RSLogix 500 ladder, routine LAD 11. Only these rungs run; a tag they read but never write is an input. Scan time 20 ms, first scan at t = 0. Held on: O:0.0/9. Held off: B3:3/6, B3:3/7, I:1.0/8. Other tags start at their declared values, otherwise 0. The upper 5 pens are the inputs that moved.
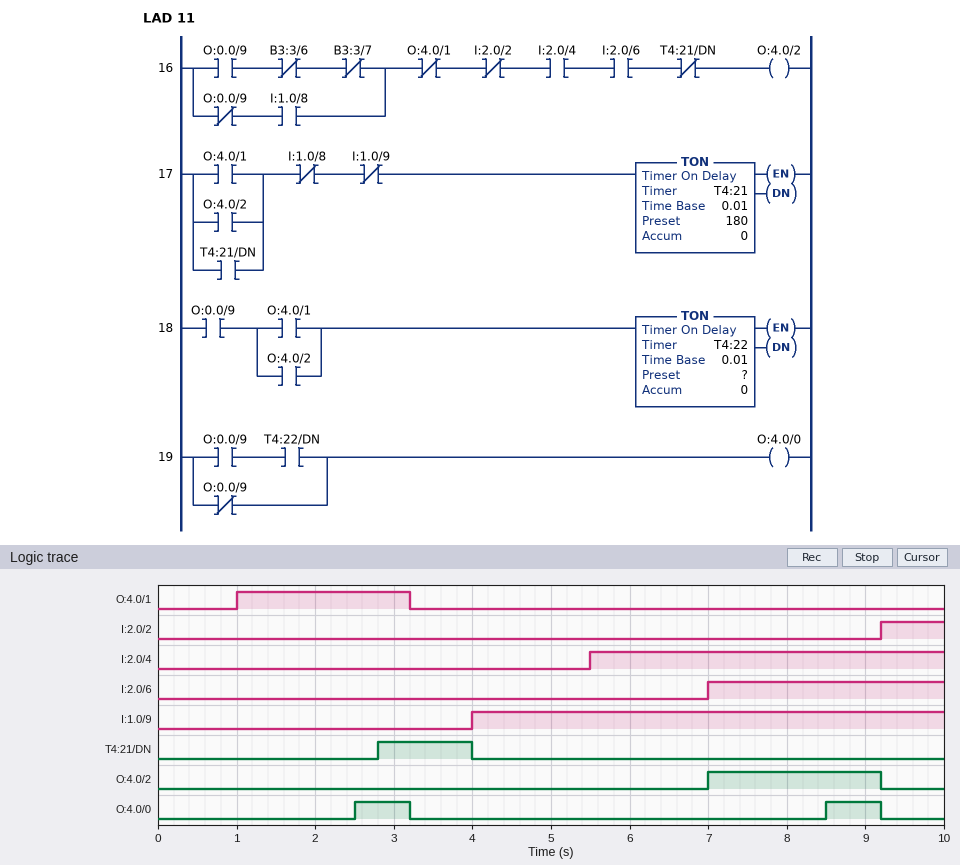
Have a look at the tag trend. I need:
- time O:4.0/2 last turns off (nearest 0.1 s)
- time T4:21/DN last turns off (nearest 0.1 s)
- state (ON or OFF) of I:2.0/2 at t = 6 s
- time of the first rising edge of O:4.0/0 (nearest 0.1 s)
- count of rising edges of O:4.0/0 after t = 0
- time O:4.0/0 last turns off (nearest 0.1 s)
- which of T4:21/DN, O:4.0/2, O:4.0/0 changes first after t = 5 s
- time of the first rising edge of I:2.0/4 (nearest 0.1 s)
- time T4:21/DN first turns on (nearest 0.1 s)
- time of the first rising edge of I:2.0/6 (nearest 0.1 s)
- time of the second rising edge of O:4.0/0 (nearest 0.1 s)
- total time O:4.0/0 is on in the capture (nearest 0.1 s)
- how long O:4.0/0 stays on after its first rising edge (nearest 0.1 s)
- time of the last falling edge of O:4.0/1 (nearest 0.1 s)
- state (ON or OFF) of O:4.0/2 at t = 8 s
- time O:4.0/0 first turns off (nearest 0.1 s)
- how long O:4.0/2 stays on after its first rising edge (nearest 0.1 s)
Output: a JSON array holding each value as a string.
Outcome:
["9.2 s", "4.0 s", "OFF", "2.5 s", "2", "9.2 s", "O:4.0/2", "5.5 s", "2.8 s", "7.0 s", "8.5 s", "1.4 s", "0.7 s", "3.2 s", "ON", "3.2 s", "2.2 s"]
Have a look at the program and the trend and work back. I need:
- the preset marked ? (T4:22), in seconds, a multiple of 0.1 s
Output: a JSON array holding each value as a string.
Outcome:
["1.5 s"]
